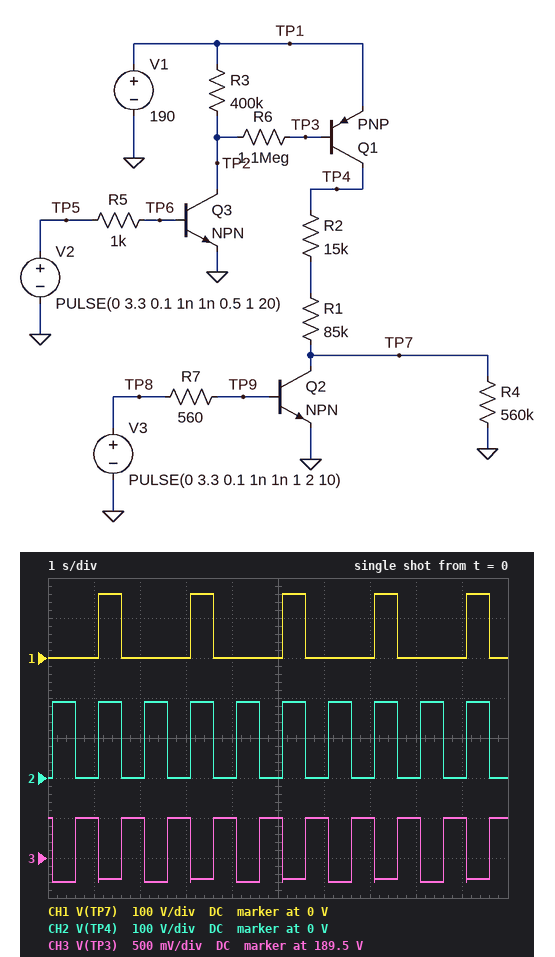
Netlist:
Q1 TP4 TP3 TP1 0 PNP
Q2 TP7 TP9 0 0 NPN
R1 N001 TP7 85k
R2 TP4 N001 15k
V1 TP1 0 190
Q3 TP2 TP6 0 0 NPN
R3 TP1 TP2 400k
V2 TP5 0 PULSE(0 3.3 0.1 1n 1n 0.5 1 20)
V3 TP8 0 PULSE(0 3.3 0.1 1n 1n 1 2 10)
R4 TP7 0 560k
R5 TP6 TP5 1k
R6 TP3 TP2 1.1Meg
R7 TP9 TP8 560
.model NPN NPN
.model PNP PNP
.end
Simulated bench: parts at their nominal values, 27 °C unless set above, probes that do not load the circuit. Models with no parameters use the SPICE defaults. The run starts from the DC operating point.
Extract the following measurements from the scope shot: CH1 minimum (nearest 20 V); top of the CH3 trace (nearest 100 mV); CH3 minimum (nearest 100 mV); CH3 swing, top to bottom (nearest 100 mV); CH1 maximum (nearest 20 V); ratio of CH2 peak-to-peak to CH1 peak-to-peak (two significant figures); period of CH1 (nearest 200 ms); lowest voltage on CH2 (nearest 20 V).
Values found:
0 V
190.0 V
189.2 V
800 mV
160 V
1.2
2.0 s
0 V
